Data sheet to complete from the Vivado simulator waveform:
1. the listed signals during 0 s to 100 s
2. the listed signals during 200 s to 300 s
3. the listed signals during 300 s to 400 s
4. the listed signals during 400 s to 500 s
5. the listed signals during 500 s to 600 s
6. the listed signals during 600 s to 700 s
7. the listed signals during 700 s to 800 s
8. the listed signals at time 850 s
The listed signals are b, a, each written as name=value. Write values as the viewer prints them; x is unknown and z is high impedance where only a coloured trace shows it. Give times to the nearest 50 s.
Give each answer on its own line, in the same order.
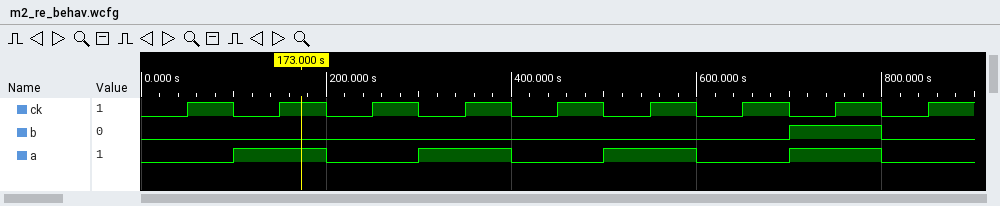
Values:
b=0, a=0
b=0, a=0
b=0, a=1
b=0, a=0
b=0, a=1
b=0, a=0
b=1, a=1
b=0, a=0
